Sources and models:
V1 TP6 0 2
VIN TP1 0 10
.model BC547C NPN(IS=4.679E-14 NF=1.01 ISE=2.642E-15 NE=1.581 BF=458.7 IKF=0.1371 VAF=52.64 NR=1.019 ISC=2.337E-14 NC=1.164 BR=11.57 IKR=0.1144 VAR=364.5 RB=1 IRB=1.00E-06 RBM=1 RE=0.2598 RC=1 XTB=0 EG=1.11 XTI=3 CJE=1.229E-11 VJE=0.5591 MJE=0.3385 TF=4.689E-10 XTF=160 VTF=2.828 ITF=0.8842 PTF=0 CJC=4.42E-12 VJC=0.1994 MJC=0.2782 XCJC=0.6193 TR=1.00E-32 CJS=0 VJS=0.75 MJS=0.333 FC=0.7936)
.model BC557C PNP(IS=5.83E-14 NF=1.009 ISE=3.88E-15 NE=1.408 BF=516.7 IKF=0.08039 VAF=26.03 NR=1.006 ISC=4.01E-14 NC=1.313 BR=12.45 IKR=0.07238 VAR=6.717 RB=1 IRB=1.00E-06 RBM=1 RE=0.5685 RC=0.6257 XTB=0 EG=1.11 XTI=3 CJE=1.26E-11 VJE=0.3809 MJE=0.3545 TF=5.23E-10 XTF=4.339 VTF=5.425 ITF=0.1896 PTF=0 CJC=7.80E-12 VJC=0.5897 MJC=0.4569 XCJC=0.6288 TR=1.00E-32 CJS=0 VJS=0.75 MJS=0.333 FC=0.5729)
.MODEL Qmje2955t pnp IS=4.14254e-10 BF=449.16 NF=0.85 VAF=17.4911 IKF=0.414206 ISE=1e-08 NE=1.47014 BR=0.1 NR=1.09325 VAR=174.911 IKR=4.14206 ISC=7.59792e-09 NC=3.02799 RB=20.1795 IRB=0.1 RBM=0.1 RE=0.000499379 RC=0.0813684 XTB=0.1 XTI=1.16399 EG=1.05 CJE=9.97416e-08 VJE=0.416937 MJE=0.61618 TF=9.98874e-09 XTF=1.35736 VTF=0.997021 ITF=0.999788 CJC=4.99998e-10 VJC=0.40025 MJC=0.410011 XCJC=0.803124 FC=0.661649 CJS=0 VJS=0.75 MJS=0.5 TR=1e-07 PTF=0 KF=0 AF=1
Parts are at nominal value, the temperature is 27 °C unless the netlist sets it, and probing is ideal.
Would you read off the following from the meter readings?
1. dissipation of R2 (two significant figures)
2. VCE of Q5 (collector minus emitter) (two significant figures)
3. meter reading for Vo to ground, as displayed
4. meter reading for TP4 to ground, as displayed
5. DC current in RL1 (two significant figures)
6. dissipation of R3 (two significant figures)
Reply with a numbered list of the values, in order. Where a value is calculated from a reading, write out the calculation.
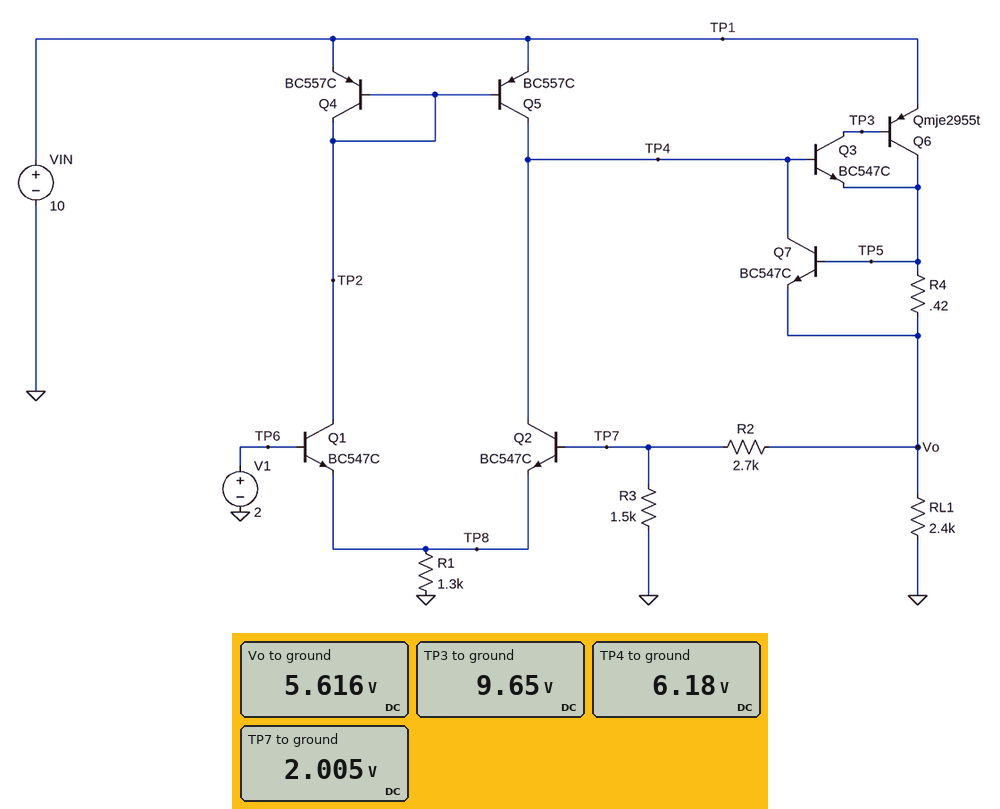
1. (5.616 V - 2.005 V)^2 / 2.7 kΩ = 4.8 mW
2. 6.18 V - 10 V = -3.8 V
3. 5.616 V
4. 6.18 V
5. (5.616 V) / 2.4 kΩ = 2.3 mA
6. (2.005 V)^2 / 1.5 kΩ = 2.7 mW
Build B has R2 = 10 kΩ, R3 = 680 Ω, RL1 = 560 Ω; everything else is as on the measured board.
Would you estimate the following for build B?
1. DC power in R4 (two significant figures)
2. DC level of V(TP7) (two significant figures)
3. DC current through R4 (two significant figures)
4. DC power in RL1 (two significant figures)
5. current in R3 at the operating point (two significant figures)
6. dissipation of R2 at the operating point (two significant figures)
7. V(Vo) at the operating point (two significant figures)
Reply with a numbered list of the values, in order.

1. 130 µW
2. 600 mV
3. 18 mA
4. 160 mW
5. 880 µA
6. 7.7 mW
7. 9.4 V
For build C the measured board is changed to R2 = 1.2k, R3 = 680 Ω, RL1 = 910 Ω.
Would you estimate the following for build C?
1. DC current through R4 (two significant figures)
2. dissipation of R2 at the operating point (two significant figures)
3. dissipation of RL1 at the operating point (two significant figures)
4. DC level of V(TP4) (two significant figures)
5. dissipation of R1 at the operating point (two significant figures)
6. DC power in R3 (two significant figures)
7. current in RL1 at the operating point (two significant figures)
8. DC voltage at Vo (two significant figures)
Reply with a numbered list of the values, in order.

1. 9.0 mA
2. 10 mW
3. 34 mW
4. 6.1 V
5. 1.5 mW
6. 5.9 mW
7. 6.1 mA
8. 5.5 V
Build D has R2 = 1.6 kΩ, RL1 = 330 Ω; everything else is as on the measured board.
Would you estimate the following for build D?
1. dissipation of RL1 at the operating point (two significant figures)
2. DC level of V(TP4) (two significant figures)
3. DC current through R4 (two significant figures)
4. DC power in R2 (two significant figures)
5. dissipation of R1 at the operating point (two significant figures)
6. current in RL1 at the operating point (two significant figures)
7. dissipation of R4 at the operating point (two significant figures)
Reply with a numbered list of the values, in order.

1. 52 mW
2. 4.7 V
3. 14 mA
4. 2.9 mW
5. 1.5 mW
6. 13 mA
7. 81 µW
